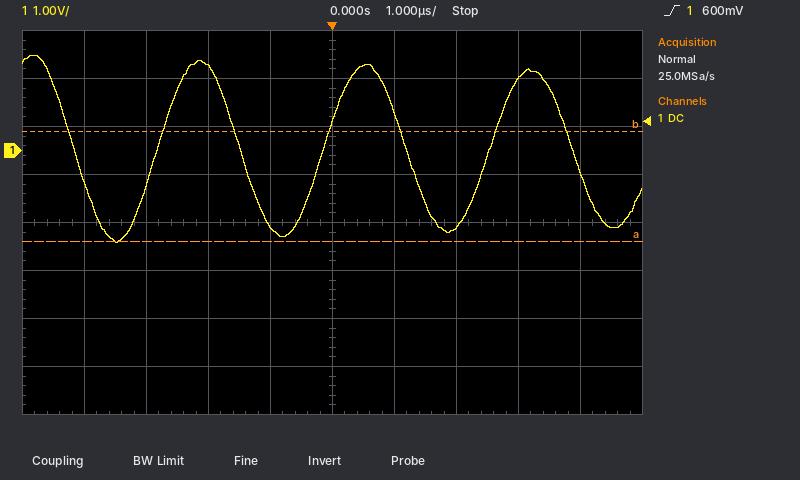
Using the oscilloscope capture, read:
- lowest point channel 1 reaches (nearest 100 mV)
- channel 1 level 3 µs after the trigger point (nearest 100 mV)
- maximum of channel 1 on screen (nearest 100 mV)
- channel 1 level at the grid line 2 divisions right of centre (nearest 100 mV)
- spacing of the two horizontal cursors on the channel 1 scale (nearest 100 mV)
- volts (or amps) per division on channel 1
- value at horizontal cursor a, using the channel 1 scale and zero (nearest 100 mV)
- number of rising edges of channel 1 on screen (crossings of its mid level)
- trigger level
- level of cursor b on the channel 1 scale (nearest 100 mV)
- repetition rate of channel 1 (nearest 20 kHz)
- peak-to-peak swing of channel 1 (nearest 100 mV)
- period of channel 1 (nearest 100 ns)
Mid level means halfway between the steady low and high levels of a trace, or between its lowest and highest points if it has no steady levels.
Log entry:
-1.9 V
1.5 V
2.0 V
-1.6 V
2.3 V
1 V
-1.9 V
3
600 mV
400 mV
380 kHz
3.9 V
2.7 µs
